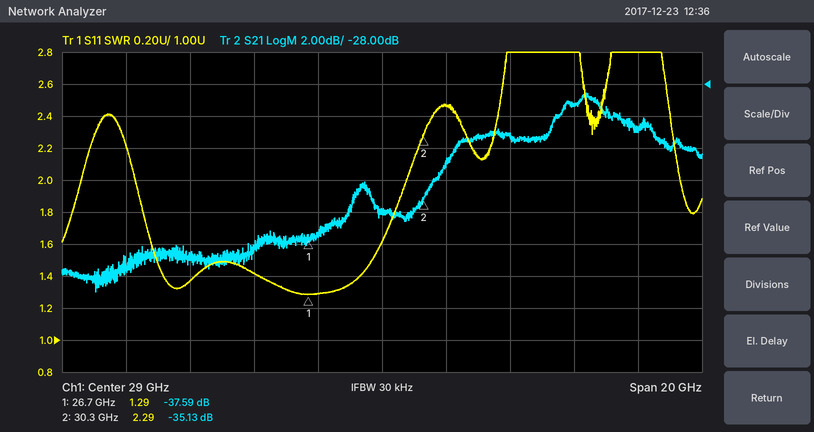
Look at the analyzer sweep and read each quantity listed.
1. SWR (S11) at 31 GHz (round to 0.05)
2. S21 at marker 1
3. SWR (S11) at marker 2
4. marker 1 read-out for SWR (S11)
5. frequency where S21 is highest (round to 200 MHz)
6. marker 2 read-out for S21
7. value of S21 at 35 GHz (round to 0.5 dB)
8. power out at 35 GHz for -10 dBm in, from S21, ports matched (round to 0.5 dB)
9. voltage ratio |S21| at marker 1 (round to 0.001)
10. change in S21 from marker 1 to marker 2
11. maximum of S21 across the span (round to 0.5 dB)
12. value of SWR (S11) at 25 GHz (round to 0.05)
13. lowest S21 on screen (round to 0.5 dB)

2.45
-37.59 dB
2.29
1.29
35.4 GHz
-35.13 dB
-29.5 dB
-39.5 dBm
0.013
2.46 dB
-28.5 dB
1.40
-41.0 dB
